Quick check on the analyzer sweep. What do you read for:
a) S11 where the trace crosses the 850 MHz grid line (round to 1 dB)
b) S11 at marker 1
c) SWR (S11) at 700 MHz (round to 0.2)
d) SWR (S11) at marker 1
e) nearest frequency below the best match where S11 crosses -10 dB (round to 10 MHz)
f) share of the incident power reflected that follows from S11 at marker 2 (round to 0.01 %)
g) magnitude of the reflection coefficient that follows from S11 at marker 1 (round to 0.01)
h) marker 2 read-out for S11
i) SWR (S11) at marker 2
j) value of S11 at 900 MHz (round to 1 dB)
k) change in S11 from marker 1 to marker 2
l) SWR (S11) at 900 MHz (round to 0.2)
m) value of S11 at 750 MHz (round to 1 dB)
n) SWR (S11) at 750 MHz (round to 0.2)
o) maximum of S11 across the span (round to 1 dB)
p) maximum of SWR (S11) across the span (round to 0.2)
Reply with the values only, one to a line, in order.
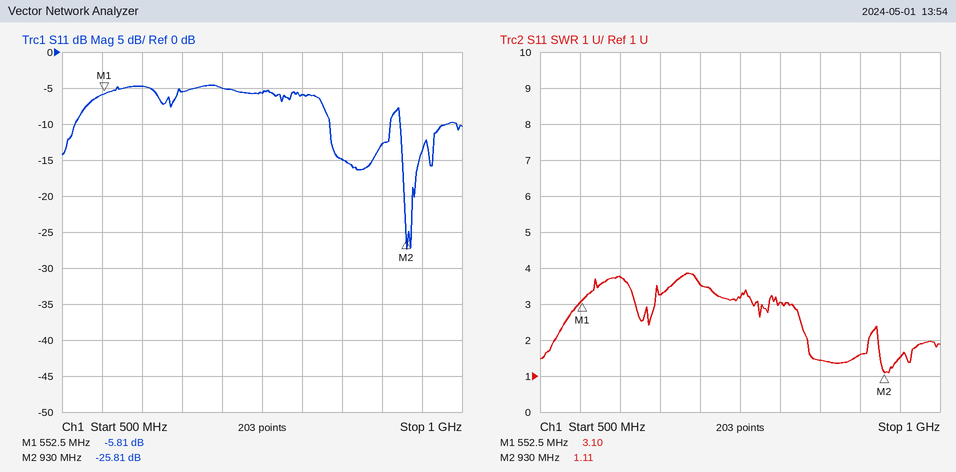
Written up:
-15 dB
-5.81 dB
3.6
3.10
920 MHz
0.26 %
0.51
-25.81 dB
1.11
-13 dB
-20.00 dB
1.6
-6 dB
3.2
-5 dB
3.8
